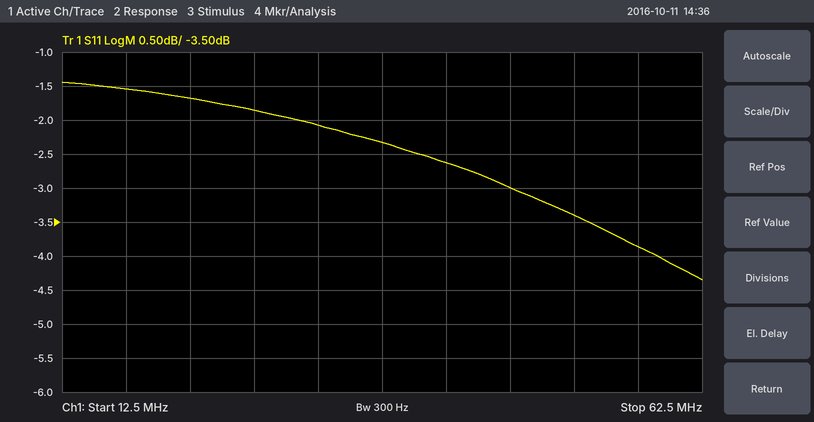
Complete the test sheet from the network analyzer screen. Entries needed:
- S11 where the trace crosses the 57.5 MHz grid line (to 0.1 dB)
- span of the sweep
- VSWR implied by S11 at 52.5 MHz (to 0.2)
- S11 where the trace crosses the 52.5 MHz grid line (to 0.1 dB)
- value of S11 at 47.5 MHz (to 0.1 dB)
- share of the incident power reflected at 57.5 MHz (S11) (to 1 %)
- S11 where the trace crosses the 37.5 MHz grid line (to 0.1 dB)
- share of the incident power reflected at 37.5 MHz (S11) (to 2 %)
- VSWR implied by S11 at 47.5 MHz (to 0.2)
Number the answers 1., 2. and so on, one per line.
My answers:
1. -3.9 dB
2. 50 MHz
3. 5.2
4. -3.4 dB
5. -3.0 dB
6. 41 %
7. -2.3 dB
8. 58 %
9. 5.8
